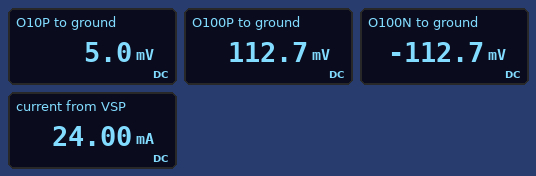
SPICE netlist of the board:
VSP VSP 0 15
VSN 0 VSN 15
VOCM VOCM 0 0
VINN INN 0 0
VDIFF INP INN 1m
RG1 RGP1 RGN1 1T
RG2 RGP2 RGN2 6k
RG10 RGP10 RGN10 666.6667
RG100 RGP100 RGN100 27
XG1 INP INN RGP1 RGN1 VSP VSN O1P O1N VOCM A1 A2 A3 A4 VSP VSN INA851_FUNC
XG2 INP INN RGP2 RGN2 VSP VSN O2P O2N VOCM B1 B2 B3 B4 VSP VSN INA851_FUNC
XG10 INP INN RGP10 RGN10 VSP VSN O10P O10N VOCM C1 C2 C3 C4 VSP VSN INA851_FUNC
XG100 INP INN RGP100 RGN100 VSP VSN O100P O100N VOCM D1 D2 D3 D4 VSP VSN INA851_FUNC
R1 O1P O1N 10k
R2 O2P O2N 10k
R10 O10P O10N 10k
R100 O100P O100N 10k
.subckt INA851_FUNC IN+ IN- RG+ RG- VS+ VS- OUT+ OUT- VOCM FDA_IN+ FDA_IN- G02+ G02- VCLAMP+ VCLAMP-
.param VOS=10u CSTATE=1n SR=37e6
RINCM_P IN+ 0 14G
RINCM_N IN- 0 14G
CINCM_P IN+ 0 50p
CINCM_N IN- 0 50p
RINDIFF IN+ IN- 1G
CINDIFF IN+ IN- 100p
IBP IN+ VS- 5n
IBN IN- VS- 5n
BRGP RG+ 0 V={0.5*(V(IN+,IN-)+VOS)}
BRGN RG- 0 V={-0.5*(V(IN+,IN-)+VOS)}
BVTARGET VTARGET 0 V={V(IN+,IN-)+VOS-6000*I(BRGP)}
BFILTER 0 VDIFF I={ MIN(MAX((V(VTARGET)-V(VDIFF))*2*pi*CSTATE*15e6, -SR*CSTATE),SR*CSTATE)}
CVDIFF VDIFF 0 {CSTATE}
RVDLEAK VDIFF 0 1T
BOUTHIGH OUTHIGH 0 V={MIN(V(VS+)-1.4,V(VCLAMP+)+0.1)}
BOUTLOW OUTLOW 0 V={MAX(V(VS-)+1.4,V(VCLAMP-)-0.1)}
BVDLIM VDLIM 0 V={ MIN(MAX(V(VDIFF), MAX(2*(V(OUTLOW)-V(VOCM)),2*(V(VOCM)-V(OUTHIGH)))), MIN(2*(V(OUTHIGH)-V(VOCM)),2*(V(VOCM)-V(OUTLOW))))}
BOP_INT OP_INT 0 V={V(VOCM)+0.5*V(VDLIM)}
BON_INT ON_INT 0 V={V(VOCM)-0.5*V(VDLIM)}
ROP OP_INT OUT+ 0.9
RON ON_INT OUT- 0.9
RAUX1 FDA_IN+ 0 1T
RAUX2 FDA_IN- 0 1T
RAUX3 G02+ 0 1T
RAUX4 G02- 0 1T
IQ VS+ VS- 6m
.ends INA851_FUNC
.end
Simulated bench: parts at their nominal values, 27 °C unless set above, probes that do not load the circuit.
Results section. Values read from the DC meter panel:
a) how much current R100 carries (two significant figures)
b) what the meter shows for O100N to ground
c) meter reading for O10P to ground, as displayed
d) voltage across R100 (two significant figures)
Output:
23 µA
-112.7 mV
5.0 mV
230 mV
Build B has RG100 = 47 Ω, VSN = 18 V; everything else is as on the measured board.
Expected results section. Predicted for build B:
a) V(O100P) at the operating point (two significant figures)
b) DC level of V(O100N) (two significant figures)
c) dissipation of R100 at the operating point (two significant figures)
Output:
65 mV
-65 mV
1.7 µW
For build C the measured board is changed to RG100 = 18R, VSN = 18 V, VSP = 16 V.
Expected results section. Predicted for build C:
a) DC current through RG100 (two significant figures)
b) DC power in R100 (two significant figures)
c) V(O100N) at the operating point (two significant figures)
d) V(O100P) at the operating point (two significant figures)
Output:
56 µA
11 µW
-170 mV
170 mV
